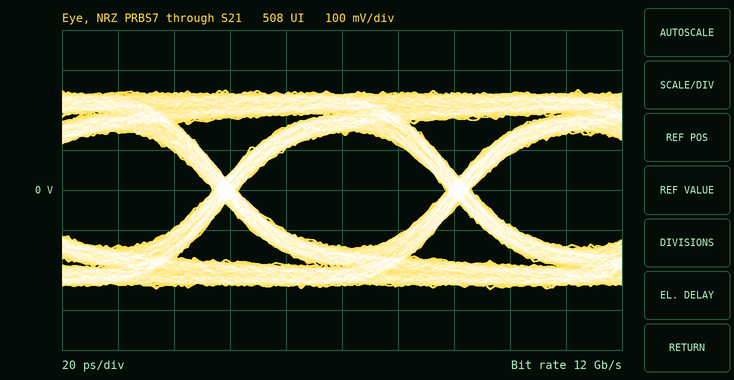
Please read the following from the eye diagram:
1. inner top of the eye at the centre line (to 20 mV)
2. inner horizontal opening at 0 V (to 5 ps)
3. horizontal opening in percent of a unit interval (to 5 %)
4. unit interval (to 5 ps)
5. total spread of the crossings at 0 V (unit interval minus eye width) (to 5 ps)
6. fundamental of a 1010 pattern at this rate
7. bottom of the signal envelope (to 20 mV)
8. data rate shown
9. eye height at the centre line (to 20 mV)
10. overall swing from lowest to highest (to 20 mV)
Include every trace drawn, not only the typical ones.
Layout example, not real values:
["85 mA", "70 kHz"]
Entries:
["140 mV", "75 ps", "90 %", "85 ps", "10 ps", "6 GHz", "-240 mV", "12 Gb/s", "280 mV", "500 mV"]
